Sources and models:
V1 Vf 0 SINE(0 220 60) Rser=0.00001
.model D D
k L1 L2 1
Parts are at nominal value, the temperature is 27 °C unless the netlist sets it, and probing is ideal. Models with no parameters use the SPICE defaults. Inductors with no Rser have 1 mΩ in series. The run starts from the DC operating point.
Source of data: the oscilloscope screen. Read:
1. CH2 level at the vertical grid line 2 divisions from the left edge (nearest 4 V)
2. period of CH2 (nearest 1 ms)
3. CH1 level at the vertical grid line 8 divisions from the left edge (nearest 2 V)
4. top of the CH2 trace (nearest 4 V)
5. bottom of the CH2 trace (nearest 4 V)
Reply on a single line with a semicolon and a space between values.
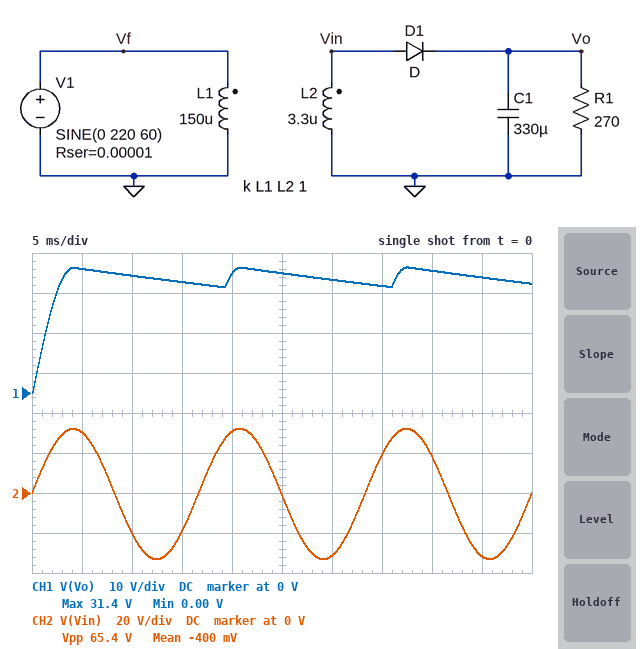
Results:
-20 V; 17 ms; 30 V; 32 V; -32 V
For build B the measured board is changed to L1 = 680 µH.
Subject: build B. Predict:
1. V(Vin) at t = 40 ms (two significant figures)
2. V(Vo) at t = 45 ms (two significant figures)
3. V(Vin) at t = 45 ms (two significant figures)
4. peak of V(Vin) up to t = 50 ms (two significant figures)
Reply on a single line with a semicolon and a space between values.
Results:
8.9 V; 13 V; -15 V; 15 V
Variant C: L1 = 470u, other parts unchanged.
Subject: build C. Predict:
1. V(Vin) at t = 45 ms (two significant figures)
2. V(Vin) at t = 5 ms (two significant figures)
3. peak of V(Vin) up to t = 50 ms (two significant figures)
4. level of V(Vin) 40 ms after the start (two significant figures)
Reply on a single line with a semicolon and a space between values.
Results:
-18 V; 17 V; 18 V; 11 V
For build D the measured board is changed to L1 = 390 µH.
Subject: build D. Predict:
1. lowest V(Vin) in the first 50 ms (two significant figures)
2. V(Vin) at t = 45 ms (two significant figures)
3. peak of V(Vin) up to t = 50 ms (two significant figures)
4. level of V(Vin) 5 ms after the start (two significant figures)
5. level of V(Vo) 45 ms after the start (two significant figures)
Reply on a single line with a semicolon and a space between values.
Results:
-20 V; -19 V; 20 V; 19 V; 18 V
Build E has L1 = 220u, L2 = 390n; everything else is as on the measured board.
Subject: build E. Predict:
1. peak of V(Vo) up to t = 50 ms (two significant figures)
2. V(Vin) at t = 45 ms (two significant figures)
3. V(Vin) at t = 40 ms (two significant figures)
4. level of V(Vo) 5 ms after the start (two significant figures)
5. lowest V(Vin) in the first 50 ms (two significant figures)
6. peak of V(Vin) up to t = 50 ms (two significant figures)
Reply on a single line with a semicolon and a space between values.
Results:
8.4 V; -8.9 V; 5.3 V; 8.3 V; -9.4 V; 9.2 V
